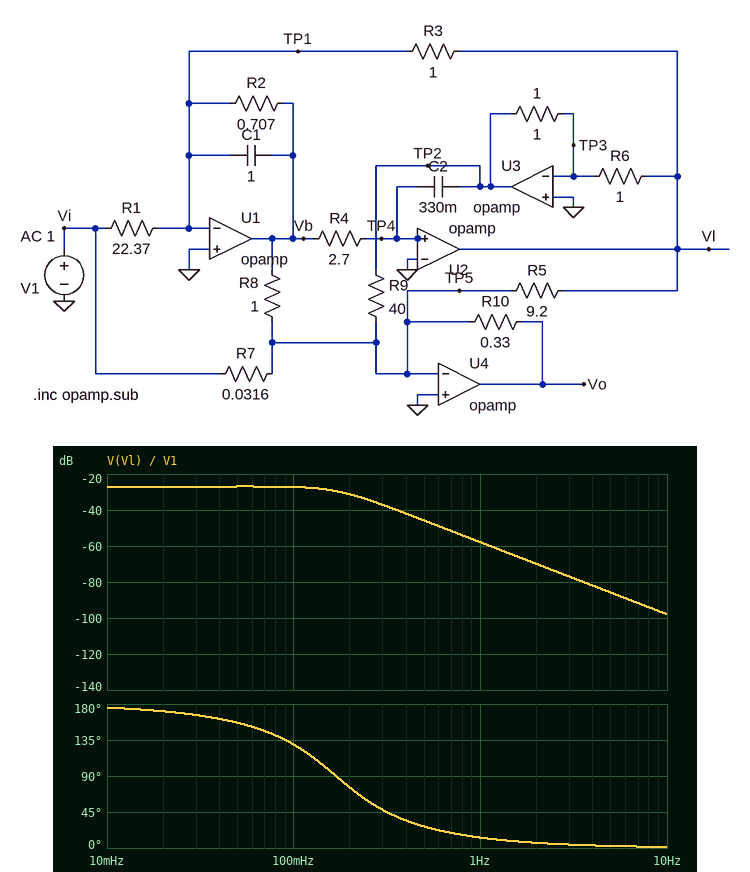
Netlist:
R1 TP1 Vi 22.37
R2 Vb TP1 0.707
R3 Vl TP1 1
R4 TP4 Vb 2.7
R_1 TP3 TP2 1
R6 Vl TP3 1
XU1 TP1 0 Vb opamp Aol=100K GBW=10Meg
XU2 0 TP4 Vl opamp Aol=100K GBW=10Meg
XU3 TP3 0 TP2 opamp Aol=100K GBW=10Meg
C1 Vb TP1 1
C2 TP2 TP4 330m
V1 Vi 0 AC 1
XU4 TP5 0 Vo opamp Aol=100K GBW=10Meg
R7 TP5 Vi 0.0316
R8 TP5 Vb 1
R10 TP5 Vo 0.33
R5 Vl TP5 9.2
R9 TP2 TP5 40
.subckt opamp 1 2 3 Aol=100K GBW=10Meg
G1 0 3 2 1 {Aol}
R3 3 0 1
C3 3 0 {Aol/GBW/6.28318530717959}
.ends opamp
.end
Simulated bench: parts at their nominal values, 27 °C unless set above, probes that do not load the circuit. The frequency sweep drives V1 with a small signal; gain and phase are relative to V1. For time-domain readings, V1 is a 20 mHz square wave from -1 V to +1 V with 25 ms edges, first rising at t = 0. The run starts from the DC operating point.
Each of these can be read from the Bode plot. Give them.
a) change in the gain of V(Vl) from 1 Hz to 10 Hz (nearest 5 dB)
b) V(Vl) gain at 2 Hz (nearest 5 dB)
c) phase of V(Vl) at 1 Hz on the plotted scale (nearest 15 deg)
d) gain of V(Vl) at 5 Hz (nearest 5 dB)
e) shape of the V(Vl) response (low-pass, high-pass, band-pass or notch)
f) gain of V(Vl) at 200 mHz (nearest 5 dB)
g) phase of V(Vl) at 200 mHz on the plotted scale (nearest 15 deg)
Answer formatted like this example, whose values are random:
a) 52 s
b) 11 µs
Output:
a) -40 dB
b) -70 dB
c) 15 deg
d) -85 dB
e) low-pass
f) -30 dB
g) 75 deg
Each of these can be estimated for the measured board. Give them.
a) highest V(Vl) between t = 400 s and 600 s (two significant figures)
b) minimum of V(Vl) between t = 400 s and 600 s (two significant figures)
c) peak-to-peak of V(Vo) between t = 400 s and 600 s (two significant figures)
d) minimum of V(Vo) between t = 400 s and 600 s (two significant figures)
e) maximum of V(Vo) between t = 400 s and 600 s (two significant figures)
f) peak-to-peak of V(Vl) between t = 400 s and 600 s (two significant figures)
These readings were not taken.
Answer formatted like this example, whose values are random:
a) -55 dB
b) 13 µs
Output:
a) 50 mV
b) -50 mV
c) 21 V
d) -10 V
e) 10 V
f) 100 mV
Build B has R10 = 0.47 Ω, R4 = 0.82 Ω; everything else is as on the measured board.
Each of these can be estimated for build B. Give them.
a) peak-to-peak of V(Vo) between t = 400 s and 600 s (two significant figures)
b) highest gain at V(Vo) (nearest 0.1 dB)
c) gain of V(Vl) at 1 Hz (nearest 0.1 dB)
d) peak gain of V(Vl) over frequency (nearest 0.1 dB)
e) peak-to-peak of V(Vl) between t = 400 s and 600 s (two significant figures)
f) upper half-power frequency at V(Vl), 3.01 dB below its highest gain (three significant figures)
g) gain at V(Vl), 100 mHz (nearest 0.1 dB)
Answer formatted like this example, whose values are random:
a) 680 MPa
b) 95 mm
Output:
a) 30 V
b) 23.4 dB
c) -47.0 dB
d) -23.7 dB
e) 140 mV
f) 364 mHz
g) -26.3 dB
